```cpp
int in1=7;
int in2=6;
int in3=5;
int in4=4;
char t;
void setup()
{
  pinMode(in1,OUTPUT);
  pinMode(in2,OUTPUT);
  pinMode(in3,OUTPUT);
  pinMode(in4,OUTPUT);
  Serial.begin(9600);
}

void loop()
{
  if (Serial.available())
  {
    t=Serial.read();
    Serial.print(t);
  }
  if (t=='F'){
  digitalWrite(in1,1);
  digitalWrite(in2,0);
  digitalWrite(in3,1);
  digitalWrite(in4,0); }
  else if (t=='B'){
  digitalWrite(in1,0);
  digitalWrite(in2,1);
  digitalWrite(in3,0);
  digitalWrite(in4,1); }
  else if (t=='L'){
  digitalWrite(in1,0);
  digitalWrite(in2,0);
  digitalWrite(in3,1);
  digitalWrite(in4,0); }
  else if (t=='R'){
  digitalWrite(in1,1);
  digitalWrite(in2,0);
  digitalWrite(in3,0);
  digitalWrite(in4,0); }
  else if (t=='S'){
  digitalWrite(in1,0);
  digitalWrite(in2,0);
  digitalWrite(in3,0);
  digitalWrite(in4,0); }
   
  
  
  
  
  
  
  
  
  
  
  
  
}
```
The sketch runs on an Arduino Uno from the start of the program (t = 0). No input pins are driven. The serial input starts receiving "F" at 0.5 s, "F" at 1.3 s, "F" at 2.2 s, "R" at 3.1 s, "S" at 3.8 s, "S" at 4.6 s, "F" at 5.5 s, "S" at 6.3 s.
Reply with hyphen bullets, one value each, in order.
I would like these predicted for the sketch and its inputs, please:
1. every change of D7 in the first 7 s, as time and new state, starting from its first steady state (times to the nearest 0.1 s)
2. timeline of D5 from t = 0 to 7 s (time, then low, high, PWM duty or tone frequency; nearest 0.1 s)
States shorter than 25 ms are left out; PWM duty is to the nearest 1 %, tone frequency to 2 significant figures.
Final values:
- 0 s low; 0.5 s high; 3.8 s low; 5.5 s high; 6.3 s low
- 0 s low; 0.5 s high; 3.1 s low; 5.5 s high; 6.3 s low
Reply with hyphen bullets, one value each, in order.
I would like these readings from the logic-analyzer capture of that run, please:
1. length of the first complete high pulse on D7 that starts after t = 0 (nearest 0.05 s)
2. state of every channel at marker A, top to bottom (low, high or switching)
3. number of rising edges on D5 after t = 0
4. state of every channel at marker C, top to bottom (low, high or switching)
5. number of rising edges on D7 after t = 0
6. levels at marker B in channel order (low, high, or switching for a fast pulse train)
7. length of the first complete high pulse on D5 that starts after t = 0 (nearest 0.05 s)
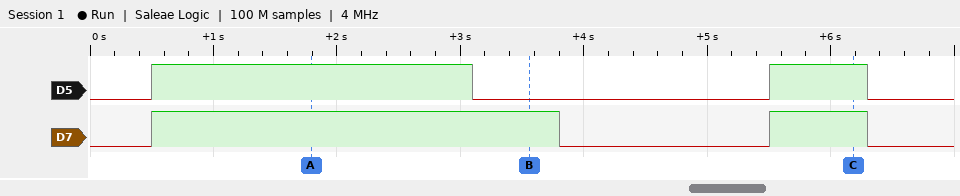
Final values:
- 3.30 s
- D5 high, D7 high
- 2
- D5 high, D7 high
- 2
- D5 low, D7 high
- 2.60 s
